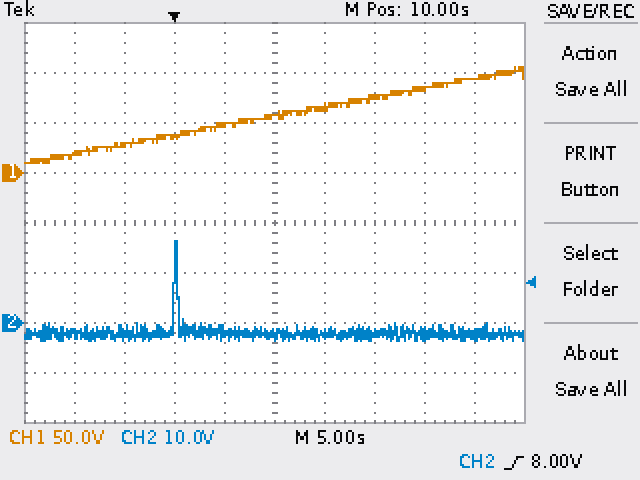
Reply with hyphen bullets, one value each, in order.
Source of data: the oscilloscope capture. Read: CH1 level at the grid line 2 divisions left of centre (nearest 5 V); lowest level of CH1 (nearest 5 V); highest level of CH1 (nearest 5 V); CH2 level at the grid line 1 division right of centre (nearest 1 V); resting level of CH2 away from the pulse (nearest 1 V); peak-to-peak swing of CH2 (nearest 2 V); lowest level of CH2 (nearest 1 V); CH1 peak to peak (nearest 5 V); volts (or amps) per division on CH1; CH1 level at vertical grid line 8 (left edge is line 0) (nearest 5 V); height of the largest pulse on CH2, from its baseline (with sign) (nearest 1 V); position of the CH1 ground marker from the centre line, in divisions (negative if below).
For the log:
- 35 V
- 10 V
- 105 V
- -2 V
- -2 V
- 20 V
- -4 V
- 95 V
- 50 V
- 85 V
- +19 V
- +1.0 div
